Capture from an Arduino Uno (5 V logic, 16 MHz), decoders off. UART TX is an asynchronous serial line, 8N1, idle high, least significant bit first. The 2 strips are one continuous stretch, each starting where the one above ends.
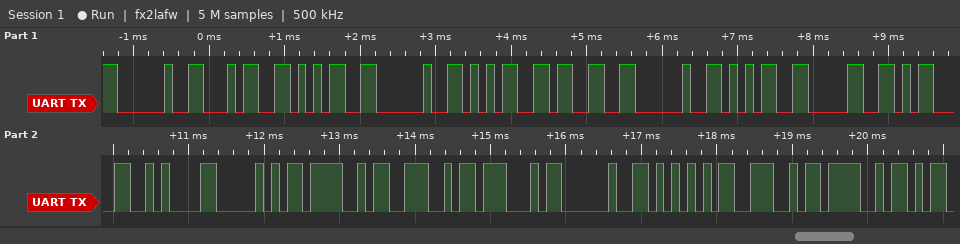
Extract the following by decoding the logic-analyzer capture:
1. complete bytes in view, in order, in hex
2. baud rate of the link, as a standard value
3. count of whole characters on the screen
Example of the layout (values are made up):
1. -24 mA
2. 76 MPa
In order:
1. 0x20 0x34 0x35 0x20 0x35 0x33 0x20 0x35 0x30 0x0D 0x0A 0x50 0x4F 0x4E 0x47 0x20 0x55 0x4E 0x4F
2. 9600 baud
3. 19
